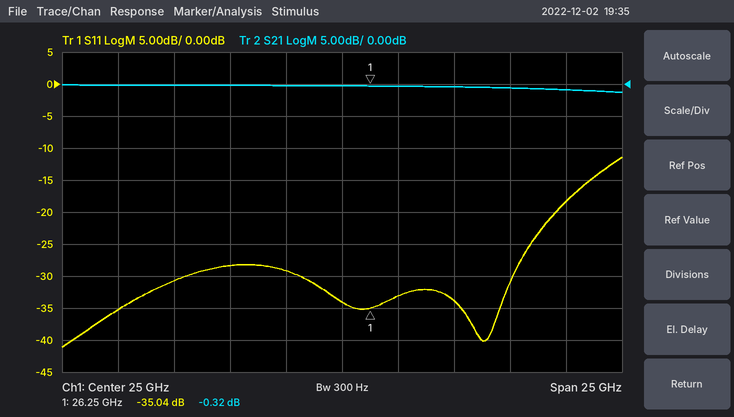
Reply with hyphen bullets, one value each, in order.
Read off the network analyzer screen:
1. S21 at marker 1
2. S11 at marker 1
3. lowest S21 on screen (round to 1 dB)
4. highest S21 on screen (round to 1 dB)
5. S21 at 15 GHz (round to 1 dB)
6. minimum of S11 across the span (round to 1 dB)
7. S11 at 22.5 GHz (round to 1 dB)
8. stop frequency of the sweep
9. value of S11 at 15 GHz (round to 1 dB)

- -0.32 dB
- -35.04 dB
- -1 dB
- 0 dB
- 0 dB
- -41 dB
- -29 dB
- 37.5 GHz
- -35 dB
